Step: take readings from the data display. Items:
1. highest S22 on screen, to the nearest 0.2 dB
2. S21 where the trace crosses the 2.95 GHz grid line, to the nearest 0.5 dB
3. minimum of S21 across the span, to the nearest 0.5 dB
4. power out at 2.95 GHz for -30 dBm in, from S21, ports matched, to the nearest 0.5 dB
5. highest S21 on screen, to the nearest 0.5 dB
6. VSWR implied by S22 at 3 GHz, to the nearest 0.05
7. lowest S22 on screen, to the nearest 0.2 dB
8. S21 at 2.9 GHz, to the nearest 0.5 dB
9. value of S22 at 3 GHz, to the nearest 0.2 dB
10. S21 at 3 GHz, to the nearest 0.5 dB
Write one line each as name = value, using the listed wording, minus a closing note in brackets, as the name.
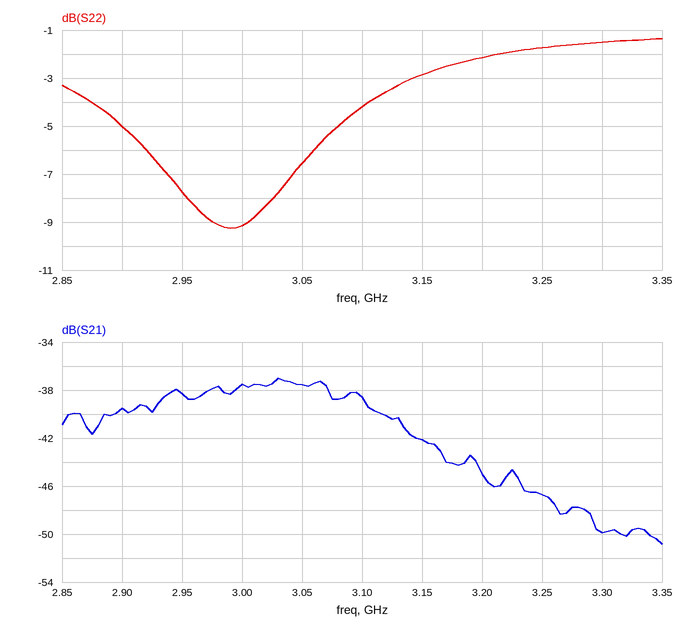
highest S22 on screen, to the nearest 0.2 dB = -1.4 dB
S21 where the trace crosses the 2.95 GHz grid line, to the nearest 0.5 dB = -38.5 dB
minimum of S21 across the span, to the nearest 0.5 dB = -51.0 dB
power out at 2.95 GHz for -30 dBm in, from S21, ports matched, to the nearest 0.5 dB = -68.5 dBm
highest S21 on screen, to the nearest 0.5 dB = -37.0 dB
VSWR implied by S22 at 3 GHz, to the nearest 0.05 = 2.05
lowest S22 on screen, to the nearest 0.2 dB = -9.2 dB
S21 at 2.9 GHz, to the nearest 0.5 dB = -39.5 dB
value of S22 at 3 GHz, to the nearest 0.2 dB = -9.2 dB
S21 at 3 GHz, to the nearest 0.5 dB = -37.5 dB
